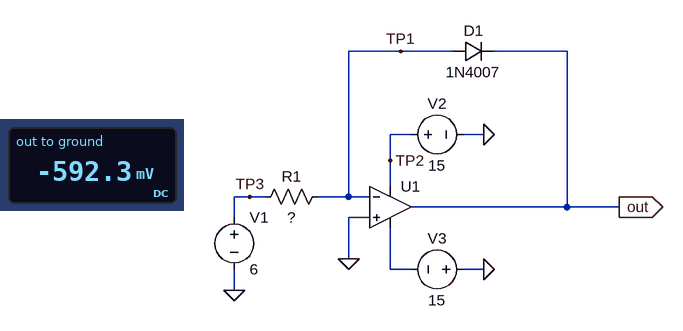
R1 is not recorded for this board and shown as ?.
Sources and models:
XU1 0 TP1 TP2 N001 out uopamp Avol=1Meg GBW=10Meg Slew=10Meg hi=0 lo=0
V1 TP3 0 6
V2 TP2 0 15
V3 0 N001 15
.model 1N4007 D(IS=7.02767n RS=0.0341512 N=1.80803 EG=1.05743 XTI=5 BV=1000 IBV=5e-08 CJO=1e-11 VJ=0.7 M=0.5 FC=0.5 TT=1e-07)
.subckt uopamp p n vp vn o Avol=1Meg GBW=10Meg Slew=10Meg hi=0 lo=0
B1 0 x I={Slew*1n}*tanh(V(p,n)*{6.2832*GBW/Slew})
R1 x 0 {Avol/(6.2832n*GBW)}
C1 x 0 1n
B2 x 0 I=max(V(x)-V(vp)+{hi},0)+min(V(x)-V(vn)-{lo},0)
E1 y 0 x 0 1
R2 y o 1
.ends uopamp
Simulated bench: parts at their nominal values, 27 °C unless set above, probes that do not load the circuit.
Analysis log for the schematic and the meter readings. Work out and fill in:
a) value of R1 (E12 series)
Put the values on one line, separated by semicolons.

2.7 kΩ
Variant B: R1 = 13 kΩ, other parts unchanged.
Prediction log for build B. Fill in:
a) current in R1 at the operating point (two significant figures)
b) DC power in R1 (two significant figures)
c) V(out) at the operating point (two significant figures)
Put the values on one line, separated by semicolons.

460 µA; 2.8 mW; -520 mV
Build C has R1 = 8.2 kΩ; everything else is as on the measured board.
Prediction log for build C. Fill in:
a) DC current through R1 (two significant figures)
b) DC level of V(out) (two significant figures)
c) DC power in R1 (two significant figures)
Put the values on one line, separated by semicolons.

730 µA; -540 mV; 4.4 mW
